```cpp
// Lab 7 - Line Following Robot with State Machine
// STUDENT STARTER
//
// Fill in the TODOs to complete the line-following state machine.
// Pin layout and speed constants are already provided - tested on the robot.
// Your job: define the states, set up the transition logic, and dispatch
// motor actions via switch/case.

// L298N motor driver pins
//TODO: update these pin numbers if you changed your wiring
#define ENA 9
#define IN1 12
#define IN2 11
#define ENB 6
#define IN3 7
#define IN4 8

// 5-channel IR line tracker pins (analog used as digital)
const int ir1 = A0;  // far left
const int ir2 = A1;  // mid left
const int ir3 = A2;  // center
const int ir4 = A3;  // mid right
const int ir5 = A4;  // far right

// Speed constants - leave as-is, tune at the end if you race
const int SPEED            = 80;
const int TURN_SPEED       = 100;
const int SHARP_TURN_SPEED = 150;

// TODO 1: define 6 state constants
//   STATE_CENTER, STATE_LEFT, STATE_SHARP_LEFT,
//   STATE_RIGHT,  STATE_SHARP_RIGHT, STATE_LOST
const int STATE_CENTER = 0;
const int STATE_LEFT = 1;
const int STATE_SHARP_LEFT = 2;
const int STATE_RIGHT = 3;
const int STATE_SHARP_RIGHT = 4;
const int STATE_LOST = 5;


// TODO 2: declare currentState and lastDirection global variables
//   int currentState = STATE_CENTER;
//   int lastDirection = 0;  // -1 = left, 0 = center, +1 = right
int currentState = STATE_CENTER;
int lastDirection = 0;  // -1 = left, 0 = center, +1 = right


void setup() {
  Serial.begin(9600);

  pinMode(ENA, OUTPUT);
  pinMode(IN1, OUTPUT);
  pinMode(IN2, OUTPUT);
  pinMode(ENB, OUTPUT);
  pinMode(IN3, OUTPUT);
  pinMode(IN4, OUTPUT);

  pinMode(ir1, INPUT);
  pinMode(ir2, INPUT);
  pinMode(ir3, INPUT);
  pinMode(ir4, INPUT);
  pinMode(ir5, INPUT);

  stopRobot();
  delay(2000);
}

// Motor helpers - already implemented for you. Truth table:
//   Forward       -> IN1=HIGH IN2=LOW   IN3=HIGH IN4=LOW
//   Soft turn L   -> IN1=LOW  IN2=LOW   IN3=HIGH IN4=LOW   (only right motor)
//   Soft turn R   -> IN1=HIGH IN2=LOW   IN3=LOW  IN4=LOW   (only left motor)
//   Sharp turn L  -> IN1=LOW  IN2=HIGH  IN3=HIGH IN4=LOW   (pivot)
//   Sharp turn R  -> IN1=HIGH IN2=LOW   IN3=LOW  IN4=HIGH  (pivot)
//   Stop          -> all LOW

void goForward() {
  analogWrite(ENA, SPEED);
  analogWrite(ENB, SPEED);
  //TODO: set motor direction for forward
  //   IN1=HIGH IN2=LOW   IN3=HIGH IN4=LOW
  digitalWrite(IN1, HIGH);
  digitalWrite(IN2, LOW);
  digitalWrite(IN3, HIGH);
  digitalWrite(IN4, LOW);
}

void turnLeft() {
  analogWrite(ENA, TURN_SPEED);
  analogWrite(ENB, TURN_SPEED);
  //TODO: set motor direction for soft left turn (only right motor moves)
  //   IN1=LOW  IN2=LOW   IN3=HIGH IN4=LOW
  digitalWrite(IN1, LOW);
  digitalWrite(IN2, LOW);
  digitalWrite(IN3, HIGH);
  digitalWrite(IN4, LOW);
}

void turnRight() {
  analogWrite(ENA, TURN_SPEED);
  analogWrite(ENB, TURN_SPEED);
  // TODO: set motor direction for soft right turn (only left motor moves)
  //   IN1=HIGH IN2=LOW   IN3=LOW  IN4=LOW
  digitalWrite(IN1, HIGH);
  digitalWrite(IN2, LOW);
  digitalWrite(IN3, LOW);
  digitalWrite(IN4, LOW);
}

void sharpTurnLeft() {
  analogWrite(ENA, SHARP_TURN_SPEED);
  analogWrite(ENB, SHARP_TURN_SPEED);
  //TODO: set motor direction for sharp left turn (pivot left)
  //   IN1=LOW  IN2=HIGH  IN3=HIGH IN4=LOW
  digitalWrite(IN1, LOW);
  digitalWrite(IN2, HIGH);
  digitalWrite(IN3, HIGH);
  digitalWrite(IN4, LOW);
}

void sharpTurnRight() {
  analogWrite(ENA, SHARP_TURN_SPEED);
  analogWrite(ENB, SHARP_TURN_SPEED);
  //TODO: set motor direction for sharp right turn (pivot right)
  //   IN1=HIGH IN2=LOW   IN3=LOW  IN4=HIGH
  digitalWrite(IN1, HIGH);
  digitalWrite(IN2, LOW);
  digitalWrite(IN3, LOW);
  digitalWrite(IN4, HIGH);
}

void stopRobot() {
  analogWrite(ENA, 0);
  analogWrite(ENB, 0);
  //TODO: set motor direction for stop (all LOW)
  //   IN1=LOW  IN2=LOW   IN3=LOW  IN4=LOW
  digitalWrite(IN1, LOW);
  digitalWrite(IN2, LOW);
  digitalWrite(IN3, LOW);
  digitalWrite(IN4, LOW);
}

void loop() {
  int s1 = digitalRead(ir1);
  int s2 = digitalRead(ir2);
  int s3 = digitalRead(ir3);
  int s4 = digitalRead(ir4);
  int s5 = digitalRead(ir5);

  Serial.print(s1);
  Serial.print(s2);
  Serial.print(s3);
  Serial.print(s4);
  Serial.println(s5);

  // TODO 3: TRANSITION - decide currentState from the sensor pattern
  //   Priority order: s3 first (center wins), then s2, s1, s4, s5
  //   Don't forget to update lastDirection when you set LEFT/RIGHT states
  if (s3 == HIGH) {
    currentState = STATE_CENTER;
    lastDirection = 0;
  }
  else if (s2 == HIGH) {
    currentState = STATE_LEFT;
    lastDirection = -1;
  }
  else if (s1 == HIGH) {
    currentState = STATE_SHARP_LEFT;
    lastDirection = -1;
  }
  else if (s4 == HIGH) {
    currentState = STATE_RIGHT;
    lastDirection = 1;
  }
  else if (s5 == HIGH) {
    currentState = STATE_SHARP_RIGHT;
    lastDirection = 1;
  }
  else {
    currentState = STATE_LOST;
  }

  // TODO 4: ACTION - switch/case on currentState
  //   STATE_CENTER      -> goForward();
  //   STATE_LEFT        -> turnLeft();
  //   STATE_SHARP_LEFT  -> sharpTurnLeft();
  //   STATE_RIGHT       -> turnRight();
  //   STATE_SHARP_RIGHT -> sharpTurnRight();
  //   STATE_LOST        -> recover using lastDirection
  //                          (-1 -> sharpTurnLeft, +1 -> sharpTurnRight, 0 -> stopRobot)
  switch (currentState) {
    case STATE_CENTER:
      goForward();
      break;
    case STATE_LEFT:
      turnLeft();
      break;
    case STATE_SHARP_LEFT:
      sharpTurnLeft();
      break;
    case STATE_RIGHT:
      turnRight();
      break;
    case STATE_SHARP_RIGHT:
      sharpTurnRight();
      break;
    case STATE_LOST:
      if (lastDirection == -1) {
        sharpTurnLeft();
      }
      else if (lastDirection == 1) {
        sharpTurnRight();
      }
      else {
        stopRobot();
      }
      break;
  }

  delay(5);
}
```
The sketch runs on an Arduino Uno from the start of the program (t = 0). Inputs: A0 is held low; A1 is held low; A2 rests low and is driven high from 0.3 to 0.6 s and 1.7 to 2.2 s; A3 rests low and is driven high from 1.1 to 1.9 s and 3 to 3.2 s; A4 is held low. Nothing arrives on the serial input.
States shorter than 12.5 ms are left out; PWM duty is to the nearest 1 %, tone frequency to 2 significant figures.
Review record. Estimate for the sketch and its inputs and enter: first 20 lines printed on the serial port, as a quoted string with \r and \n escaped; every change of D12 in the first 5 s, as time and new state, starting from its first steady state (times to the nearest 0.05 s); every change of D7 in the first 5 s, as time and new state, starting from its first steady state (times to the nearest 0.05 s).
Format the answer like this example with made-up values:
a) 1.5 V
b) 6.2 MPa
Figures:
a) "00100\r\n00100\r\n00100\r\n00100\r\n00100\r\n00100\r\n00100\r\n00100\r\n00100\r\n00100\r\n00100\r\n00100\r\n00100\r\n00100\r\n00100\r\n00100\r\n00100\r\n00100\r\n00100\r\n00100\r\n"
b) 0 s low; 2 s high; 2.2 s low; 3 s high
c) 0 s low; 2 s high; 2.2 s low
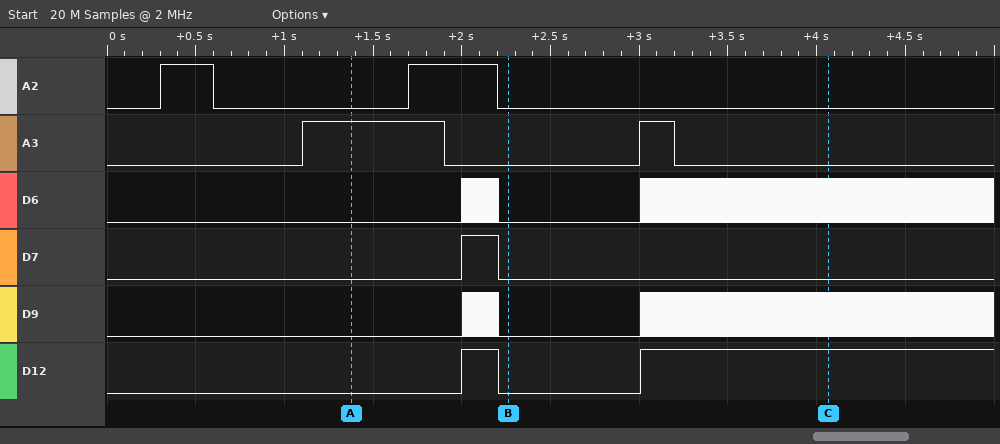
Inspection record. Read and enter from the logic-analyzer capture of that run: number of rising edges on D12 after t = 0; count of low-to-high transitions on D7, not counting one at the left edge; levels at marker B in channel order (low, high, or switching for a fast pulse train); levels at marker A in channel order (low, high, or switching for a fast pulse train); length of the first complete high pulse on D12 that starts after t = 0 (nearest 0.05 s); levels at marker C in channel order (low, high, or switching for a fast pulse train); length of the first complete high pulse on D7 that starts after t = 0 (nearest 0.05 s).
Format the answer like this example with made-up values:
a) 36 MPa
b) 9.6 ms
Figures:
a) 2
b) 1
c) A2 low, A3 low, D6 low, D7 low, D9 low, D12 low
d) A2 low, A3 high, D6 low, D7 low, D9 low, D12 low
e) 0.20 s
f) A2 low, A3 low, D6 switching, D7 low, D9 switching, D12 high
g) 0.20 s
